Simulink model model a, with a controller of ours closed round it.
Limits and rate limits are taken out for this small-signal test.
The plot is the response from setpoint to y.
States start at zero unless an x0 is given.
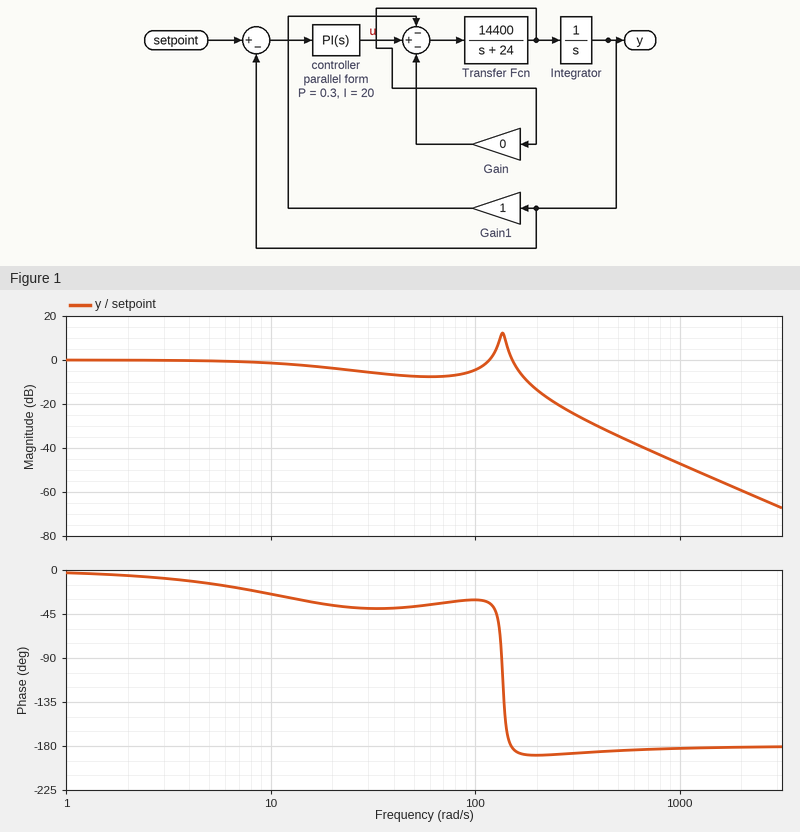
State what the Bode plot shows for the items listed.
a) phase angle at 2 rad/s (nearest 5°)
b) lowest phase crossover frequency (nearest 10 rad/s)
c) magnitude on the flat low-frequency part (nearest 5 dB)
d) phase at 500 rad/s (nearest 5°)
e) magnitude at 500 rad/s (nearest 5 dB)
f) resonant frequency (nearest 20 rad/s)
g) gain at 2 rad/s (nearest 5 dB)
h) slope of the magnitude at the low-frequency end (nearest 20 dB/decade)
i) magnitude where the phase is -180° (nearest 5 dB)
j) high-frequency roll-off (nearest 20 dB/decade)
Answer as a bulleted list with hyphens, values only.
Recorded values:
- -5°
- 150 rad/s
- 0 dB
- -185°
- -35 dB
- 140 rad/s
- 0 dB
- 0 dB/decade
- 0 dB
- -40 dB/decade
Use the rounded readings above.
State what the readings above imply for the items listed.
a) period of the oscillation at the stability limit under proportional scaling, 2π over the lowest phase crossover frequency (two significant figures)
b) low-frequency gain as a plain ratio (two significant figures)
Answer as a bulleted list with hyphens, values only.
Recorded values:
- 0.042 s
- 1.0
